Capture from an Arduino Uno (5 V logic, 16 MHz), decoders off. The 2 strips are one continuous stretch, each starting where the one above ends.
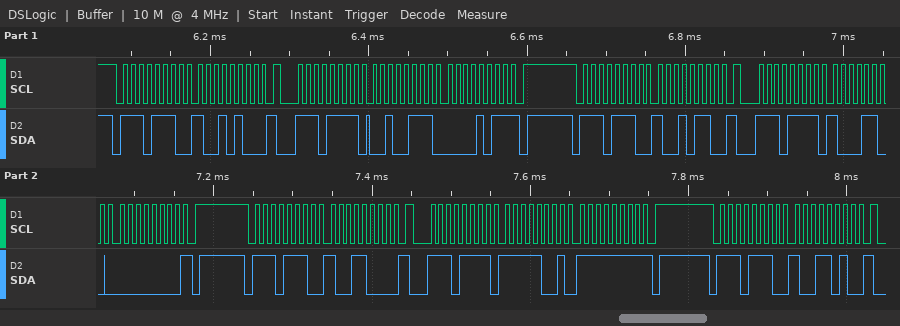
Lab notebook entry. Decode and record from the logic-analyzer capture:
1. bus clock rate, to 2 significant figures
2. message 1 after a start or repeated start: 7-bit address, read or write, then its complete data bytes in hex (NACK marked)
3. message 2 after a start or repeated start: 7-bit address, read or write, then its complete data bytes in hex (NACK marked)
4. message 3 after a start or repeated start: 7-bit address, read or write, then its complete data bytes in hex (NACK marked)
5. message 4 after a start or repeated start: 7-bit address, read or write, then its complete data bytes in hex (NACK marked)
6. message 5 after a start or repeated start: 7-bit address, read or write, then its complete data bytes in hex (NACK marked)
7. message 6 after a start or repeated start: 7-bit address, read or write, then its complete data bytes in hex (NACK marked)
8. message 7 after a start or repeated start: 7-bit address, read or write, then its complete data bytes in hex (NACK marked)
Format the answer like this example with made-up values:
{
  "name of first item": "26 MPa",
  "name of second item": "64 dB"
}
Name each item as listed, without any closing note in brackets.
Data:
{
  "bus clock rate, to 2 significant figures": "100 kHz",
  "message 1 after a start or repeated start: 7-bit address, read or write, then its complete data bytes in hex": "0x77 write: 94",
  "message 2 after a start or repeated start: 7-bit address, read or write, then its complete data bytes in hex": "0x77 read: 27 0B NACK",
  "message 3 after a start or repeated start: 7-bit address, read or write, then its complete data bytes in hex": "0x77 write: 96",
  "message 4 after a start or repeated start: 7-bit address, read or write, then its complete data bytes in hex": "0x77 read: 8C 00 NACK",
  "message 5 after a start or repeated start: 7-bit address, read or write, then its complete data bytes in hex": "0x77 write: 98",
  "message 6 after a start or repeated start: 7-bit address, read or write, then its complete data bytes in hex": "0x77 read: F9 FF NACK",
  "message 7 after a start or repeated start: 7-bit address, read or write, then its complete data bytes in hex": "0x77 write: 9A"
}
